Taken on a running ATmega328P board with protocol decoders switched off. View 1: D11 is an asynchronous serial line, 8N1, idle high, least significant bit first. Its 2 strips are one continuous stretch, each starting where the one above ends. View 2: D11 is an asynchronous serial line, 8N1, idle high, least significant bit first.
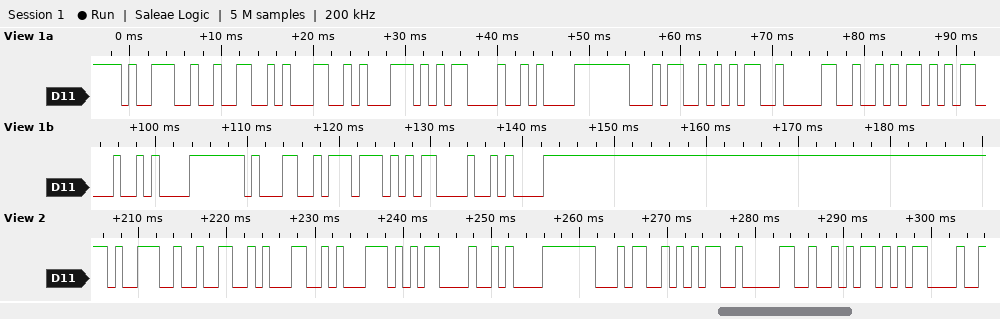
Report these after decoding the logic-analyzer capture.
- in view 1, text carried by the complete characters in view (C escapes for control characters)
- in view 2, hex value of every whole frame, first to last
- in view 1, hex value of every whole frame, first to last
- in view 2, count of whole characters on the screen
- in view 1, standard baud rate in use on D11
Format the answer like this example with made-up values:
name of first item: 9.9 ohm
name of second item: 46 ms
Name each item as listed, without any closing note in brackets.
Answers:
in view 1, text carried by the complete characters in view: "921q\r\n450j\r\n1w\r\n"
in view 2, hex value of every whole frame, first to last: 39 32 31 71 0D 0A 34 35 30 6A 0D
in view 1, hex value of every whole frame, first to last: 39 32 31 71 0D 0A 34 35 30 6A 0D 0A 31 77 0D 0A
in view 2, count of whole characters on the screen: 11
in view 1, standard baud rate in use on D11: 1200 baud
